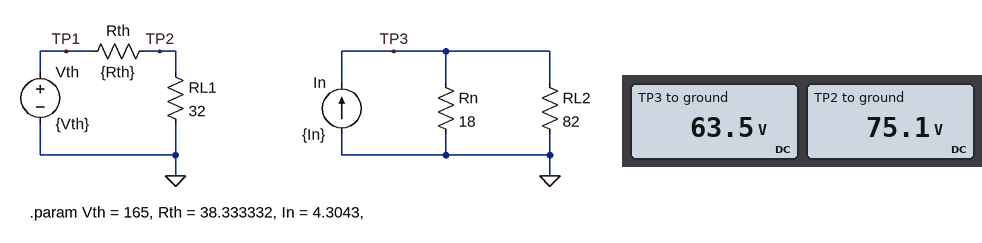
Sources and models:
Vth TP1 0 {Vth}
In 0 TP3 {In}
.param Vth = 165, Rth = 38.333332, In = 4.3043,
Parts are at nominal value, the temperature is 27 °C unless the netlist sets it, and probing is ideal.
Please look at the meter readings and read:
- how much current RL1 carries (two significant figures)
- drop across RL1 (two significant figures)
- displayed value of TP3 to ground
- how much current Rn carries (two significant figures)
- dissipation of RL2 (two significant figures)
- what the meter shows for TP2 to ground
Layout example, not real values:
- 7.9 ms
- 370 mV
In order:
- 2.3 A
- 75 V
- 63.5 V
- 3.5 A
- 49 W
- 75.1 V
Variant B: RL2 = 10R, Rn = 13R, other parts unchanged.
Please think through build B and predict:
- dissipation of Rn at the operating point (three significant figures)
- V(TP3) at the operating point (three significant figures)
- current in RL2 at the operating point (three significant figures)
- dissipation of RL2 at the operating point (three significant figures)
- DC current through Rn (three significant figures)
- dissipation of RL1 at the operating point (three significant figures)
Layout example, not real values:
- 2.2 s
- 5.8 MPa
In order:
- 45.5 W
- 24.3 V
- 2.43 A
- 59.2 W
- 1.87 A
- 176 W
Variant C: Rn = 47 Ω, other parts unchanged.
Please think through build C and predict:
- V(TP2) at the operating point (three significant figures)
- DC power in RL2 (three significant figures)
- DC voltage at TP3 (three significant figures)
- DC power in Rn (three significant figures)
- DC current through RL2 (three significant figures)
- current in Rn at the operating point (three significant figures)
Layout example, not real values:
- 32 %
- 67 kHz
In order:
- 75.1 V
- 202 W
- 129 V
- 352 W
- 1.57 A
- 2.74 A
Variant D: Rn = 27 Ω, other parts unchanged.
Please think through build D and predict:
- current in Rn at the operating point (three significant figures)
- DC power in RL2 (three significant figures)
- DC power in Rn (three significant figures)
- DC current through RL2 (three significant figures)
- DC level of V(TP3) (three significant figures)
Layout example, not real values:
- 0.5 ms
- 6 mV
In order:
- 3.24 A
- 93.2 W
- 283 W
- 1.07 A
- 87.4 V
